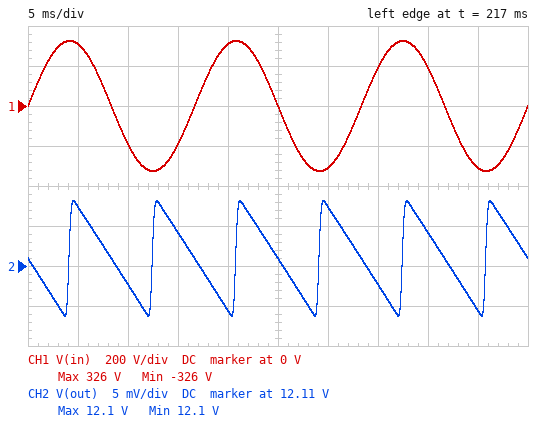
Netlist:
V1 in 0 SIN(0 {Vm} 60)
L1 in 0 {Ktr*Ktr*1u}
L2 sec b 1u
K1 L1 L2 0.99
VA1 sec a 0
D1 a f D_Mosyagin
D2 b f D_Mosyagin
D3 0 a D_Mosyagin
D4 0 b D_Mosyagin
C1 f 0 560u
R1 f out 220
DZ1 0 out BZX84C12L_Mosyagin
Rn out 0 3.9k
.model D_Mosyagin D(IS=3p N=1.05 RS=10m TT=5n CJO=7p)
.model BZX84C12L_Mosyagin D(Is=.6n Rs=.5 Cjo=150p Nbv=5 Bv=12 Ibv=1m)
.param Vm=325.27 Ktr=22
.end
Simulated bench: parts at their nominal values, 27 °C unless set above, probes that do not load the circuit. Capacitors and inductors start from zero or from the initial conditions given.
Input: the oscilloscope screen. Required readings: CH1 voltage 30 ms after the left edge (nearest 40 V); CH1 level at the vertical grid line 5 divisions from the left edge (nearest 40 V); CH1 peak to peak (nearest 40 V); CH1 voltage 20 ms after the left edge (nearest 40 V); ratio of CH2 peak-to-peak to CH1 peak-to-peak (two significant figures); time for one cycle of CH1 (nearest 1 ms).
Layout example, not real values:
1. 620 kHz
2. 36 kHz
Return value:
1. -320 V
2. 0 V
3. 640 V
4. 320 V
5. 0.000022
6. 17 ms
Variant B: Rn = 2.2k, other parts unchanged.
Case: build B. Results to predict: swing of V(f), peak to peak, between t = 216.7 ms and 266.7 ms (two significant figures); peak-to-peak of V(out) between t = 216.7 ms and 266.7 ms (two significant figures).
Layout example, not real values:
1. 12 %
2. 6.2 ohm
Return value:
1. 81 mV
2. 36 mV
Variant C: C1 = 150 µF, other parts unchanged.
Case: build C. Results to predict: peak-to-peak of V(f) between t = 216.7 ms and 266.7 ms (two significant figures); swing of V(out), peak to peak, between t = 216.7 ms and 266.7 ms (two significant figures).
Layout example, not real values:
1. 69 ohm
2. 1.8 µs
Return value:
1. 260 mV
2. 55 mV
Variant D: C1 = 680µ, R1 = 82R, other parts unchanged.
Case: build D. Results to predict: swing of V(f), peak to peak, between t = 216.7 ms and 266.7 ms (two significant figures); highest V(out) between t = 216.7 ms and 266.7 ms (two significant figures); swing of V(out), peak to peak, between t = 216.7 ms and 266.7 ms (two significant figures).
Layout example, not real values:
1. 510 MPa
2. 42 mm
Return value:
1. 130 mV
2. 12 V
3. 20 mV
